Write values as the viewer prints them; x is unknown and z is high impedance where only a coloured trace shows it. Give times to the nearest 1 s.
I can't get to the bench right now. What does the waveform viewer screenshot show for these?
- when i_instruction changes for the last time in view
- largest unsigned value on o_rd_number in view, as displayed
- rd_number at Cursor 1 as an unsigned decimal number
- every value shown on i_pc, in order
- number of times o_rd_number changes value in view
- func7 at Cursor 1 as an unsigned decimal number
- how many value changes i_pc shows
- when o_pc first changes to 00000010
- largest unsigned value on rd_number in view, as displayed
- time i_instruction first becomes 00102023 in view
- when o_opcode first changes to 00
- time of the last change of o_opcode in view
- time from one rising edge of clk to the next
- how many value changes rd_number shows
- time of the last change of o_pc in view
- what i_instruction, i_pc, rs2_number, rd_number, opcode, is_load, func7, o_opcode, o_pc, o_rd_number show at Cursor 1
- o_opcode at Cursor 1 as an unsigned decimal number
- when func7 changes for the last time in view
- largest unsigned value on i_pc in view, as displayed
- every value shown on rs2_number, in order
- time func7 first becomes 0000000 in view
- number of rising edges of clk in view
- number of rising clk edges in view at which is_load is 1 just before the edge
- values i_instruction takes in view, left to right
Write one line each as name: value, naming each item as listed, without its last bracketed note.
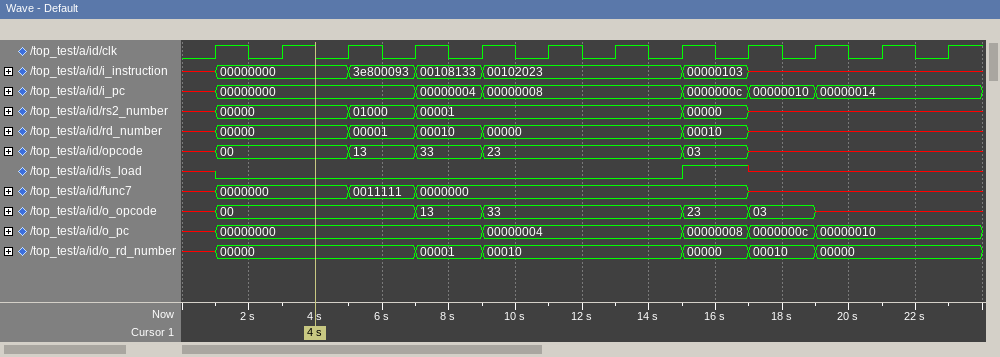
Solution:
when i_instruction changes for the last time in view: 17 s
largest unsigned value on o_rd_number in view, as displayed: 00010
rd_number at Cursor 1 as an unsigned decimal number: 0
every value shown on i_pc, in order: x, 00000000, 00000004, 00000008, 0000000c, 00000010, 00000014
number of times o_rd_number changes value in view: 6
func7 at Cursor 1 as an unsigned decimal number: 0
how many value changes i_pc shows: 6
when o_pc first changes to 00000010: 19 s
largest unsigned value on rd_number in view, as displayed: 00010
time i_instruction first becomes 00102023 in view: 9 s
when o_opcode first changes to 00: 1 s
time of the last change of o_opcode in view: 19 s
time from one rising edge of clk to the next: 2 s
how many value changes rd_number shows: 6
time of the last change of o_pc in view: 19 s
what i_instruction, i_pc, rs2_number, rd_number, opcode, is_load, func7, o_opcode, o_pc, o_rd_number show at Cursor 1: i_instruction=00000000, i_pc=00000000, rs2_number=00000, rd_number=00000, opcode=00, is_load=0, func7=0000000, o_opcode=00, o_pc=00000000, o_rd_number=00000
o_opcode at Cursor 1 as an unsigned decimal number: 0
when func7 changes for the last time in view: 17 s
largest unsigned value on i_pc in view, as displayed: 00000014
every value shown on rs2_number, in order: x, 00000, 01000, 00001, 00000, x
time func7 first becomes 0000000 in view: 1 s
number of rising edges of clk in view: 12
number of rising clk edges in view at which is_load is 1 just before the edge: 1
values i_instruction takes in view, left to right: x, 00000000, 3e800093, 00108133, 00102023, 00000103, x
